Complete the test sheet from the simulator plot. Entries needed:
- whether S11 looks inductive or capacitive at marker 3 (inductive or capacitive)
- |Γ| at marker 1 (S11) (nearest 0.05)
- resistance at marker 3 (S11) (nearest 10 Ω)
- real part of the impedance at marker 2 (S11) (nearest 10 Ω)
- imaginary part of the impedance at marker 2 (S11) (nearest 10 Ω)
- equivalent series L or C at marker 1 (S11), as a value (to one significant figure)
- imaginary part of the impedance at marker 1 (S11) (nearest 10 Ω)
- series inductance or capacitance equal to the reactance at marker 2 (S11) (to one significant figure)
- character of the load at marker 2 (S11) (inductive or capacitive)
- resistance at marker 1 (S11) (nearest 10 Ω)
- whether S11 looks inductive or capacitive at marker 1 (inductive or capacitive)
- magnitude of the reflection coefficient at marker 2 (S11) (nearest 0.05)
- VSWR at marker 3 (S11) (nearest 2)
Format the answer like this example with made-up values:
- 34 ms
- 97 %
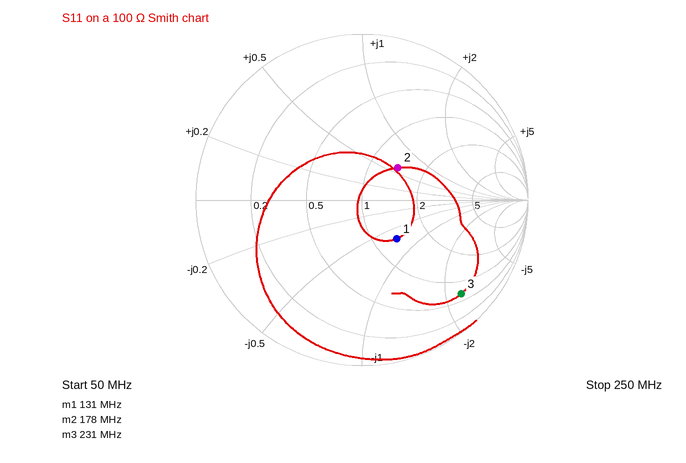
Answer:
- capacitive
- 0.30
- 70 Ω
- 140 Ω
- +60 Ω
- 20 pF
- -70 Ω
- 50 nH
- inductive
- 130 Ω
- capacitive
- 0.30
- 10
